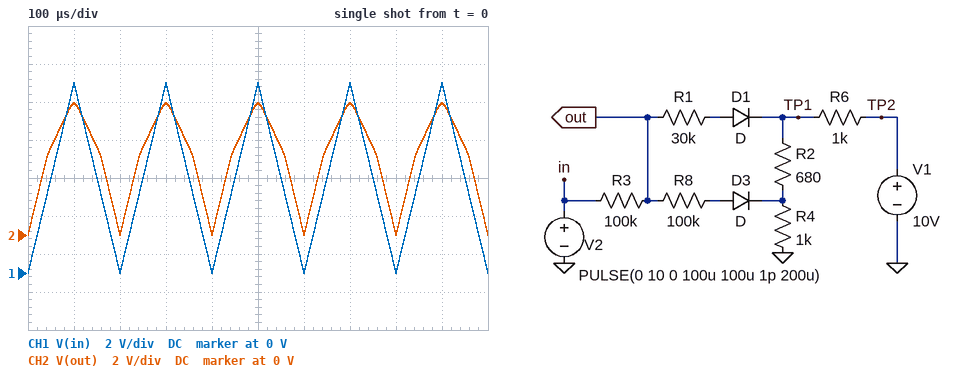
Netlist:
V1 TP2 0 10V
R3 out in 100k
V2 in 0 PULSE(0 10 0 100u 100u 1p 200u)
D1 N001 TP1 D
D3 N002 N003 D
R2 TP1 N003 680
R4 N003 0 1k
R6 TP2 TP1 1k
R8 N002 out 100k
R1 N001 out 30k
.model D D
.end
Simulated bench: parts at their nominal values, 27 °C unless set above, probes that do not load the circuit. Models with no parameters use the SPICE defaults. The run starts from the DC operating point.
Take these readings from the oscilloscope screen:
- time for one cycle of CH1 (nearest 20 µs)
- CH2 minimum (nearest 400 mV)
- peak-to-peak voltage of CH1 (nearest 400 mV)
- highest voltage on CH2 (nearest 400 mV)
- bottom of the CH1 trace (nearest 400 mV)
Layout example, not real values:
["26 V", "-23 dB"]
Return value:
["200 µs", "0 V", "10.0 V", "6.8 V", "0 V"]
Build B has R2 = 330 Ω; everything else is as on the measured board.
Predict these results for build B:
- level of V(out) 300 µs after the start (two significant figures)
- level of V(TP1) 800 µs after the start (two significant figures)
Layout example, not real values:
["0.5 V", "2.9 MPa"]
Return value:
["6.7 V", "5.7 V"]
